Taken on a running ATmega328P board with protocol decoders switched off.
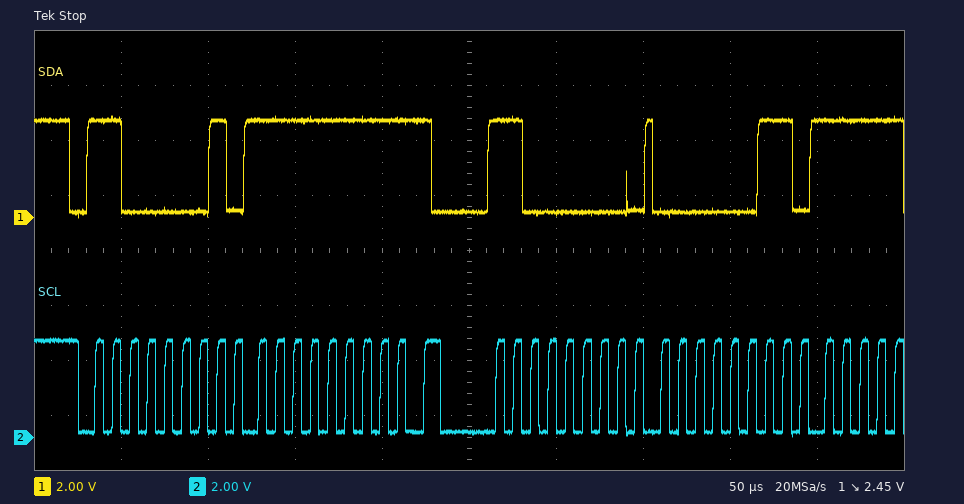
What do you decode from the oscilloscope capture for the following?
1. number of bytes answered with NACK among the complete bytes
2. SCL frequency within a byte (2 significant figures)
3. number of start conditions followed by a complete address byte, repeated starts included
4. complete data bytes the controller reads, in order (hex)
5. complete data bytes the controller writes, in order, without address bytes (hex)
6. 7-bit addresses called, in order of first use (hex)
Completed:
1
100 kHz
2
FF
03
0x60
